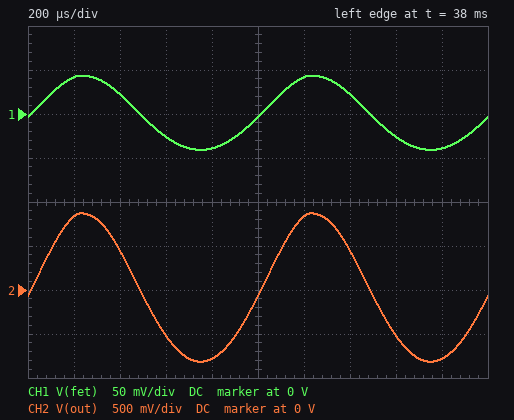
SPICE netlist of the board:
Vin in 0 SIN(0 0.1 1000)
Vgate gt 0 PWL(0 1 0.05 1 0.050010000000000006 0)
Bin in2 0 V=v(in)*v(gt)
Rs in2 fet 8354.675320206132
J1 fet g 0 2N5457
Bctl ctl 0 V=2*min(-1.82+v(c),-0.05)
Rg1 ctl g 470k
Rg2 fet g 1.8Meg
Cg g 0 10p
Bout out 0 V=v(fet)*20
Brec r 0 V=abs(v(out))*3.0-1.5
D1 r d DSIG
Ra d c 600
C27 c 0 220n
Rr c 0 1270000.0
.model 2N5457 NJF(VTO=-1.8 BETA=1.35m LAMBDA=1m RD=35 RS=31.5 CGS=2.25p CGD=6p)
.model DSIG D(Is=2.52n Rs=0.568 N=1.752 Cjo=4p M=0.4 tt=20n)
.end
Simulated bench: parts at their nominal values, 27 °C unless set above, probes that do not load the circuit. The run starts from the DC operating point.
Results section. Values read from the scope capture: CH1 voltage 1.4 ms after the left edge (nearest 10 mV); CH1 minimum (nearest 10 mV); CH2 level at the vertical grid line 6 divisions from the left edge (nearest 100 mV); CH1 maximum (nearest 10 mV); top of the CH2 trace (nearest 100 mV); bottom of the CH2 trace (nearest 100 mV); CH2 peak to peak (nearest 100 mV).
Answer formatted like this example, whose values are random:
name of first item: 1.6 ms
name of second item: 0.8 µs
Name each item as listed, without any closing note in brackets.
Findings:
CH1 voltage 1.4 ms after the left edge: 20 mV
CH1 minimum: -40 mV
CH2 level at the vertical grid line 6 divisions from the left edge: 800 mV
CH1 maximum: 40 mV
top of the CH2 trace: 900 mV
bottom of the CH2 trace: -800 mV
CH2 peak to peak: 1.7 V
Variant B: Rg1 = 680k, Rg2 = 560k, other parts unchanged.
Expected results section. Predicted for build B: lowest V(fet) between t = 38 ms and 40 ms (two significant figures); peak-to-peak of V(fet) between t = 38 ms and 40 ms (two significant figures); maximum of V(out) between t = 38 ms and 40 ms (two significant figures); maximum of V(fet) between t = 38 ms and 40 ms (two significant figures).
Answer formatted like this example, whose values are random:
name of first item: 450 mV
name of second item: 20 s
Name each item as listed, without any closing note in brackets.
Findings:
lowest V(fet) between t = 38 ms and 40 ms: -28 mV
peak-to-peak of V(fet) between t = 38 ms and 40 ms: 45 mV
maximum of V(out) between t = 38 ms and 40 ms: 340 mV
maximum of V(fet) between t = 38 ms and 40 ms: 17 mV
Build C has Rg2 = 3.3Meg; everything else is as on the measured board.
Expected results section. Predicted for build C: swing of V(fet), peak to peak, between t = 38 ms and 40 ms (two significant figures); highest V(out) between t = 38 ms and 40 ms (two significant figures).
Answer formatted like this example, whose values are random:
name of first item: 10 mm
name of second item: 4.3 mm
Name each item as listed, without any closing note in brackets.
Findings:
swing of V(fet), peak to peak, between t = 38 ms and 40 ms: 83 mV
highest V(out) between t = 38 ms and 40 ms: 910 mV
